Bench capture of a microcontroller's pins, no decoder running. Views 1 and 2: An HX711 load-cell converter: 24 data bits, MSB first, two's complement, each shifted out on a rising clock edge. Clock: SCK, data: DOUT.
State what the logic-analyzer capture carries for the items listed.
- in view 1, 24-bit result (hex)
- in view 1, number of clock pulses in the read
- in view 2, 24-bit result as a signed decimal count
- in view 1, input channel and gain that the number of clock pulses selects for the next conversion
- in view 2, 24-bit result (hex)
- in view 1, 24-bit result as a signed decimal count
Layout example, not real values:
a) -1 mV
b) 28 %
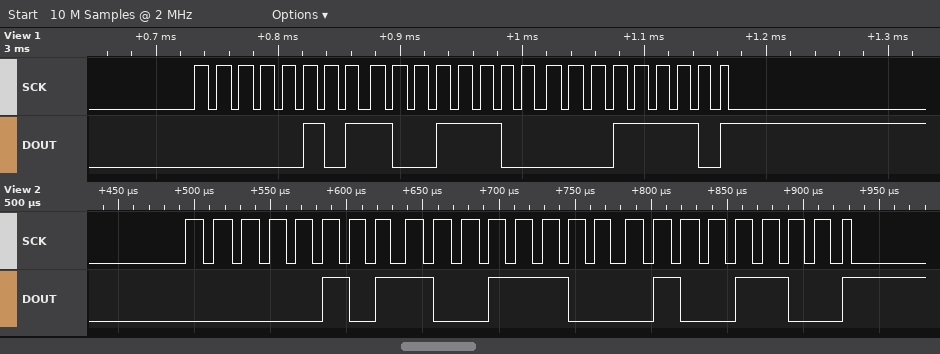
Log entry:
a) 0x059C1E
b) 25
c) 367692
d) channel A, gain 128
e) 0x059C4C
f) 367646
